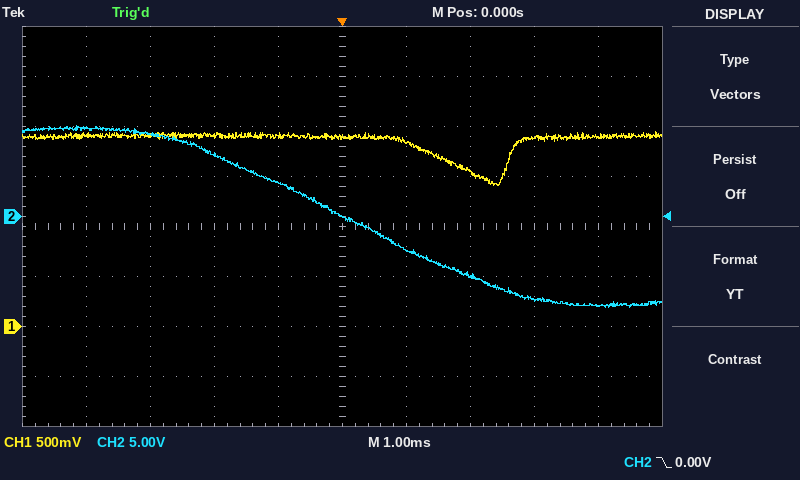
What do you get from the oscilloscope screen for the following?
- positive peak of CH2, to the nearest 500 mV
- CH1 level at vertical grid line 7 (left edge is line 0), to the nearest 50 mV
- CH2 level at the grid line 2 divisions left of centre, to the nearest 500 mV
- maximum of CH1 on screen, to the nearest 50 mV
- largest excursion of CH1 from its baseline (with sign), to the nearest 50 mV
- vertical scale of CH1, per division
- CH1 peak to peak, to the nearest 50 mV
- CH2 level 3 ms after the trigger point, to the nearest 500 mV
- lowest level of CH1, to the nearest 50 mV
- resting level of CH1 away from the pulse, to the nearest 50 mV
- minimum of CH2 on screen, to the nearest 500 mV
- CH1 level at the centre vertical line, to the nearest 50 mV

9.0 V
1.55 V
6.0 V
1.95 V
-500 mV
500 mV
550 mV
-8.5 V
1.40 V
1.90 V
-9.0 V
1.90 V
